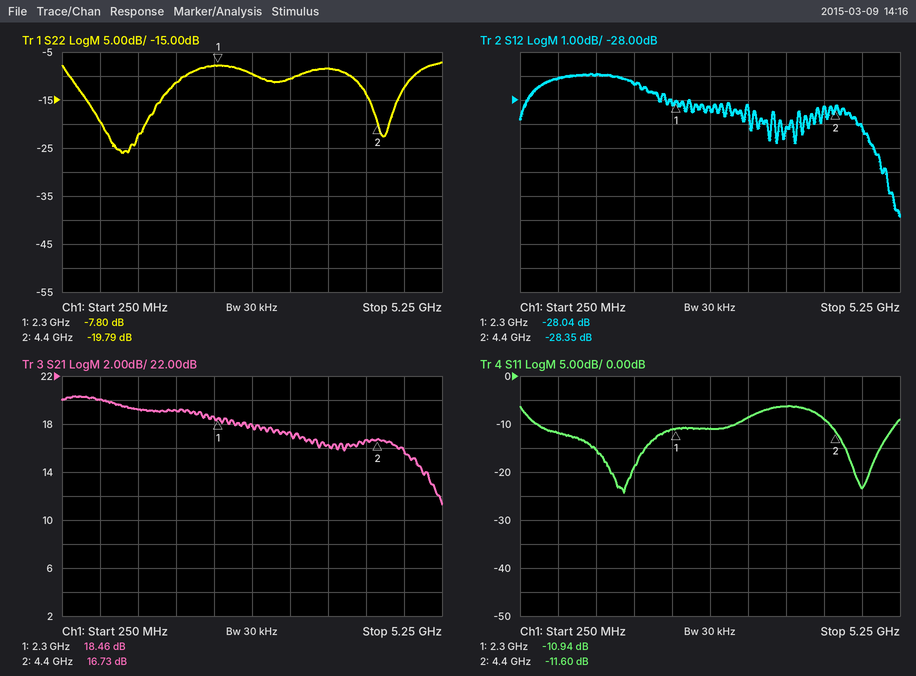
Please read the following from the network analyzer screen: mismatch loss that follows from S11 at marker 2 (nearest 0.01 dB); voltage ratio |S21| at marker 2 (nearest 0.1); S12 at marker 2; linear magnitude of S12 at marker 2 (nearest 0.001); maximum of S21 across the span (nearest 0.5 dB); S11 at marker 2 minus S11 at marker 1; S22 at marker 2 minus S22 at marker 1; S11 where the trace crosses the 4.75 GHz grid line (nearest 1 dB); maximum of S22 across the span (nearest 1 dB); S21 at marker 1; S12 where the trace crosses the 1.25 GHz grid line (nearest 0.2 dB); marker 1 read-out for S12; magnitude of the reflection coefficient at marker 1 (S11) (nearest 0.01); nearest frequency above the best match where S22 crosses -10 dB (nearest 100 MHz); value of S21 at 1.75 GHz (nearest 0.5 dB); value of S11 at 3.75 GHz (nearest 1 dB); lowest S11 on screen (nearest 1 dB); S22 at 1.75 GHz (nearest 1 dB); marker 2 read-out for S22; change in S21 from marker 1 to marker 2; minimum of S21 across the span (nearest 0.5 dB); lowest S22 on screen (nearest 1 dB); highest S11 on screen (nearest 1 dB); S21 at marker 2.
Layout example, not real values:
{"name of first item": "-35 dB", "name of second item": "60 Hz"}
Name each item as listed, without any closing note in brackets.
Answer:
{"mismatch loss that follows from S11 at marker 2": "0.31 dB", "voltage ratio |S21| at marker 2": "6.9", "S12 at marker 2": "-28.35 dB", "linear magnitude of S12 at marker 2": "0.038", "maximum of S21 across the span": "20.5 dB", "S11 at marker 2 minus S11 at marker 1": "-0.66 dB", "S22 at marker 2 minus S22 at marker 1": "-11.99 dB", "S11 where the trace crosses the 4.75 GHz grid line": "-23 dB", "maximum of S22 across the span": "-7 dB", "S21 at marker 1": "18.46 dB", "S12 where the trace crosses the 1.25 GHz grid line": "-27.0 dB", "marker 1 read-out for S12": "-28.04 dB", "magnitude of the reflection coefficient at marker 1 (S11)": "0.28", "nearest frequency above the best match where S22 crosses -10 dB": "1.9 GHz", "value of S21 at 1.75 GHz": "19.0 dB", "value of S11 at 3.75 GHz": "-6 dB", "lowest S11 on screen": "-24 dB", "S22 at 1.75 GHz": "-11 dB", "marker 2 read-out for S22": "-19.79 dB", "change in S21 from marker 1 to marker 2": "-1.73 dB", "minimum of S21 across the span": "11.5 dB", "lowest S22 on screen": "-26 dB", "highest S11 on screen": "-6 dB", "S21 at marker 2": "16.73 dB"}
